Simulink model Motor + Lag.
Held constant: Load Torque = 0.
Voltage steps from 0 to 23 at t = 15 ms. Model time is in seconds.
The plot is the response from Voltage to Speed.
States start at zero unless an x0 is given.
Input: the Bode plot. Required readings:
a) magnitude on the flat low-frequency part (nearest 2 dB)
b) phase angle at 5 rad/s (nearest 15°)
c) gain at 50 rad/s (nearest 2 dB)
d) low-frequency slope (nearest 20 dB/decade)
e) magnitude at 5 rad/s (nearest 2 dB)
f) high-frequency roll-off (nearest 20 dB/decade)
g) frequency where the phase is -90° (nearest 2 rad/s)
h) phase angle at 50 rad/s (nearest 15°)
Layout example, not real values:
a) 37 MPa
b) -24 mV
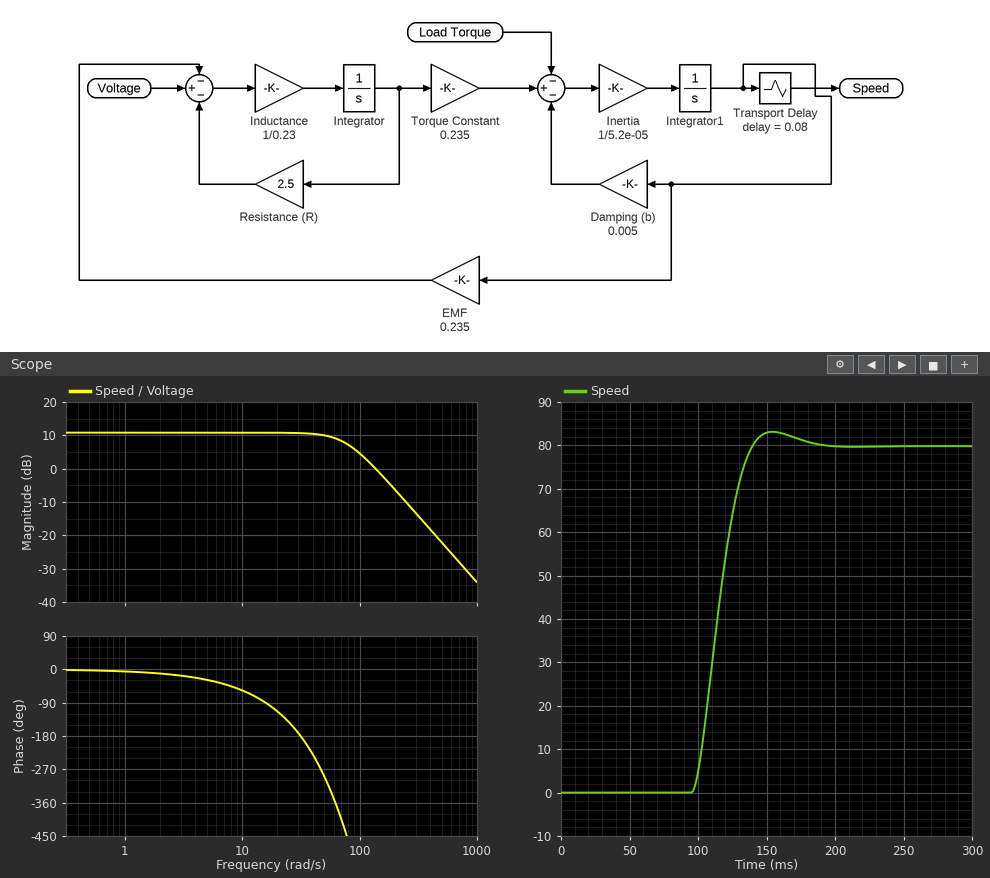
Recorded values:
a) 10 dB
b) -30°
c) 10 dB
d) 0 dB/decade
e) 10 dB
f) -40 dB/decade
g) 16 rad/s
h) -285°
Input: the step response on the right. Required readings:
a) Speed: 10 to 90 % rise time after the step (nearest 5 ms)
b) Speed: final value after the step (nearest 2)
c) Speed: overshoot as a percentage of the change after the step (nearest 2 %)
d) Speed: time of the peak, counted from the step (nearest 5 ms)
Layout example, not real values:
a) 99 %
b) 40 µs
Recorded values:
a) 30 ms
b) 80
c) 4 %
d) 140 ms
